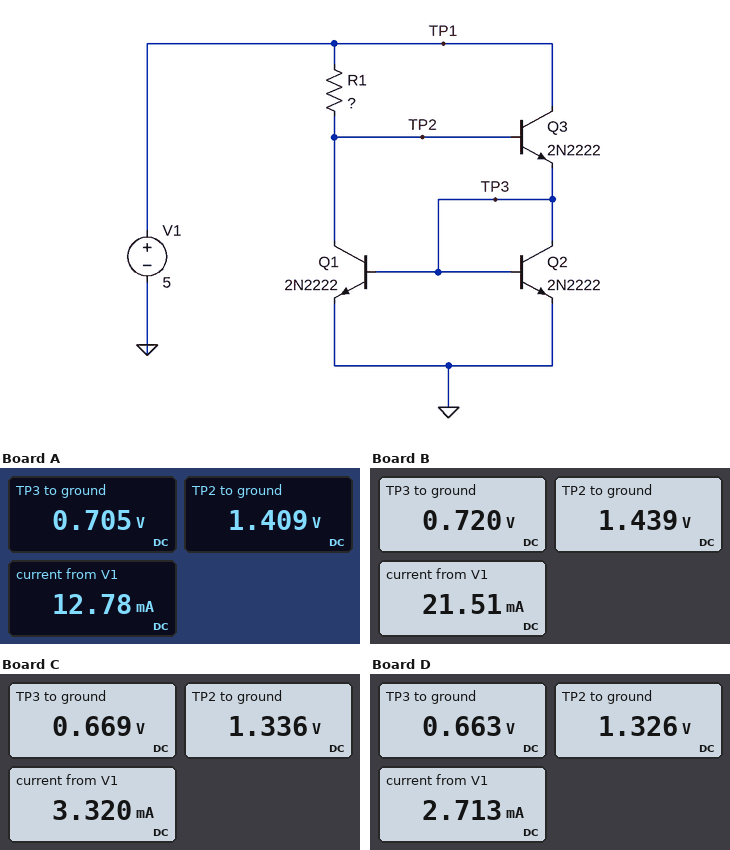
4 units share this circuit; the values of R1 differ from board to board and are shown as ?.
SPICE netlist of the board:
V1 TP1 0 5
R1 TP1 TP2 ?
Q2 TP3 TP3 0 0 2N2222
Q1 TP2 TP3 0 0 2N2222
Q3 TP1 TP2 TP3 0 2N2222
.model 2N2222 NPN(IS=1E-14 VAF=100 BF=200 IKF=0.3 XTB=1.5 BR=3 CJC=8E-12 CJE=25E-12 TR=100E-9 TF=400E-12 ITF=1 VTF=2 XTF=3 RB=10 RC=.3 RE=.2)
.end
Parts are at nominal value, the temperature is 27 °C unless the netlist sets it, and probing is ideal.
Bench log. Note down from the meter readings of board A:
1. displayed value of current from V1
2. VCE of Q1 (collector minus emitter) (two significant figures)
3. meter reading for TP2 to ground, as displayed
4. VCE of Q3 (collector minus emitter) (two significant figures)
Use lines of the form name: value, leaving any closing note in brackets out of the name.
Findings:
displayed value of current from V1: 12.78 mA
VCE of Q1 (collector minus emitter): 1.4 V
meter reading for TP2 to ground, as displayed: 1.409 V
VCE of Q3 (collector minus emitter): 4.3 V
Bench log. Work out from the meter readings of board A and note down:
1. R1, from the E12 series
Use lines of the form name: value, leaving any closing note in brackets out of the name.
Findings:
R1, from the E12 series: 560 Ω
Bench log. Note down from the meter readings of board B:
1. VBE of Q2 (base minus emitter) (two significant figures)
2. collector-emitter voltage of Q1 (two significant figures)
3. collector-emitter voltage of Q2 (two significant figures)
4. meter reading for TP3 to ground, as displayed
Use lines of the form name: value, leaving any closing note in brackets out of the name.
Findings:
VBE of Q2 (base minus emitter): 720 mV
collector-emitter voltage of Q1: 1.4 V
collector-emitter voltage of Q2: 720 mV
meter reading for TP3 to ground, as displayed: 0.720 V
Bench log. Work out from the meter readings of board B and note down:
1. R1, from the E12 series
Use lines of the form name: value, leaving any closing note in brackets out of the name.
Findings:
R1, from the E12 series: 330 Ω
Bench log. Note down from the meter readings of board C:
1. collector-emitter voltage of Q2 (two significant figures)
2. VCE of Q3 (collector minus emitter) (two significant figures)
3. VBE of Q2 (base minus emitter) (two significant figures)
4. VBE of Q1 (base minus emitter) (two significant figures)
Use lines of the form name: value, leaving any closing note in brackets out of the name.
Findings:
collector-emitter voltage of Q2: 670 mV
VCE of Q3 (collector minus emitter): 4.3 V
VBE of Q2 (base minus emitter): 670 mV
VBE of Q1 (base minus emitter): 670 mV
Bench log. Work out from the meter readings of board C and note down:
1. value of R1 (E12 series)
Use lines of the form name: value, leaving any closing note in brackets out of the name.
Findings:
value of R1: 2.2 kΩ
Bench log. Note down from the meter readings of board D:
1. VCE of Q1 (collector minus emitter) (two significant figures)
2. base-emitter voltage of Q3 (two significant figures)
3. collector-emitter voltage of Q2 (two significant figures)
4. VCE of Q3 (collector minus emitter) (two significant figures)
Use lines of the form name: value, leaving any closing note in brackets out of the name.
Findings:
VCE of Q1 (collector minus emitter): 1.3 V
base-emitter voltage of Q3: 660 mV
collector-emitter voltage of Q2: 660 mV
VCE of Q3 (collector minus emitter): 4.3 V
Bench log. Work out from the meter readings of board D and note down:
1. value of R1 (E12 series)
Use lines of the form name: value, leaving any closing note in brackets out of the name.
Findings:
value of R1: 2.7 kΩ
